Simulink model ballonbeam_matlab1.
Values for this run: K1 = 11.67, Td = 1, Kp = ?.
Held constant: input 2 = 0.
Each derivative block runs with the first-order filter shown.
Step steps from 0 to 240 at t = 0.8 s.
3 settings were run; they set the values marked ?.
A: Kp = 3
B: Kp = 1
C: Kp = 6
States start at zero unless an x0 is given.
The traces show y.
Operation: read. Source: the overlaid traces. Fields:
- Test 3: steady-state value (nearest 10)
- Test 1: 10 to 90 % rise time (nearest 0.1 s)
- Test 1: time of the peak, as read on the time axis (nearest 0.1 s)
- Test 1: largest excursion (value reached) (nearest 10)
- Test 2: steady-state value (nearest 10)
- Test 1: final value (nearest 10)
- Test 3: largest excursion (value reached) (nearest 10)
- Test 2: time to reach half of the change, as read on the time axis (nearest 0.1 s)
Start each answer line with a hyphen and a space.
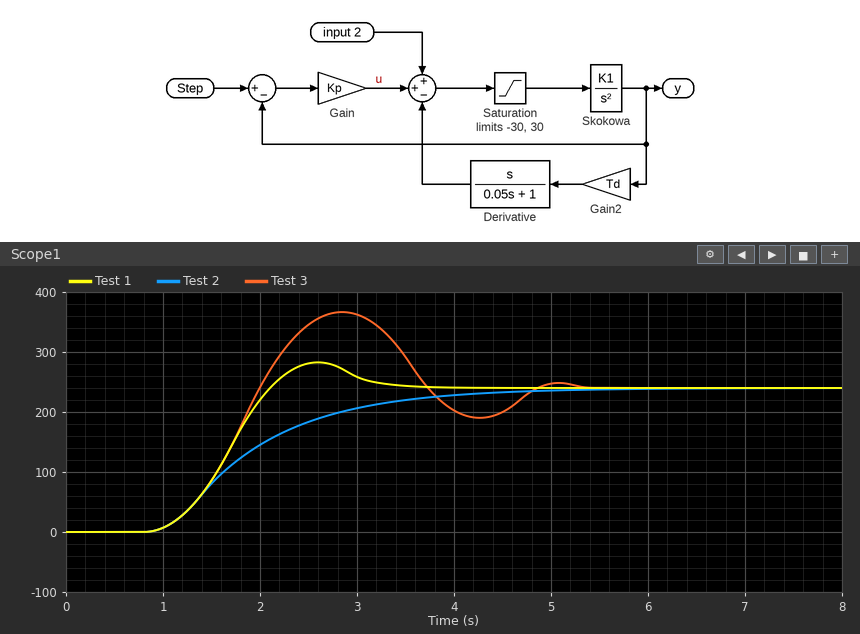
- 240
- 0.8 s
- 2.6 s
- 280
- 240
- 240
- 370
- 1.8 s
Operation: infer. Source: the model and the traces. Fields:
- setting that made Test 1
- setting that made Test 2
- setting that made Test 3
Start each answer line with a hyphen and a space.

- A
- B
- C
